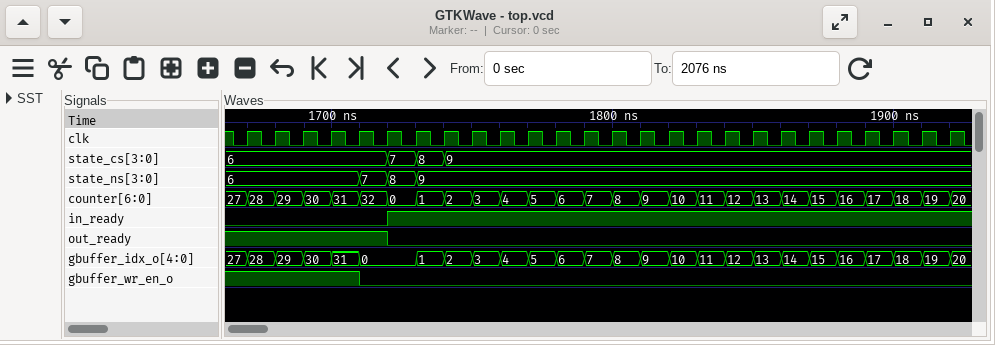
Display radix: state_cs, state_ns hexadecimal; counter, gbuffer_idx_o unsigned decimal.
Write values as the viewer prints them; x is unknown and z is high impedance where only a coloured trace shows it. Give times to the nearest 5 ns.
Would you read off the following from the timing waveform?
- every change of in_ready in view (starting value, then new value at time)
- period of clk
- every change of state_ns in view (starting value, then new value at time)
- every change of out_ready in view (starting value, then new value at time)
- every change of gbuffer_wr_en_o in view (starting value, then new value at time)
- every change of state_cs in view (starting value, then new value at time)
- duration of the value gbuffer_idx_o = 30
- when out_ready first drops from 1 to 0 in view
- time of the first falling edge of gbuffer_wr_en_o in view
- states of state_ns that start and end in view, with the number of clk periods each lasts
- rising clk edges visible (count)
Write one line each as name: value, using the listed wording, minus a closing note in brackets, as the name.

every change of in_ready in view: 0, 1 at 1720 ns
period of clk: 10 ns
every change of state_ns in view: 6, 7 at 1710 ns, 8 at 1720 ns, 9 at 1730 ns
every change of out_ready in view: 1, 0 at 1720 ns
every change of gbuffer_wr_en_o in view: 1, 0 at 1710 ns
every change of state_cs in view: 6, 7 at 1720 ns, 8 at 1730 ns, 9 at 1740 ns
duration of the value gbuffer_idx_o = 30: 10 ns
when out_ready first drops from 1 to 0 in view: 1720 ns
time of the first falling edge of gbuffer_wr_en_o in view: 1710 ns
states of state_ns that start and end in view, with the number of clk periods each lasts: 7: 1, 8: 1
rising clk edges visible: 26
